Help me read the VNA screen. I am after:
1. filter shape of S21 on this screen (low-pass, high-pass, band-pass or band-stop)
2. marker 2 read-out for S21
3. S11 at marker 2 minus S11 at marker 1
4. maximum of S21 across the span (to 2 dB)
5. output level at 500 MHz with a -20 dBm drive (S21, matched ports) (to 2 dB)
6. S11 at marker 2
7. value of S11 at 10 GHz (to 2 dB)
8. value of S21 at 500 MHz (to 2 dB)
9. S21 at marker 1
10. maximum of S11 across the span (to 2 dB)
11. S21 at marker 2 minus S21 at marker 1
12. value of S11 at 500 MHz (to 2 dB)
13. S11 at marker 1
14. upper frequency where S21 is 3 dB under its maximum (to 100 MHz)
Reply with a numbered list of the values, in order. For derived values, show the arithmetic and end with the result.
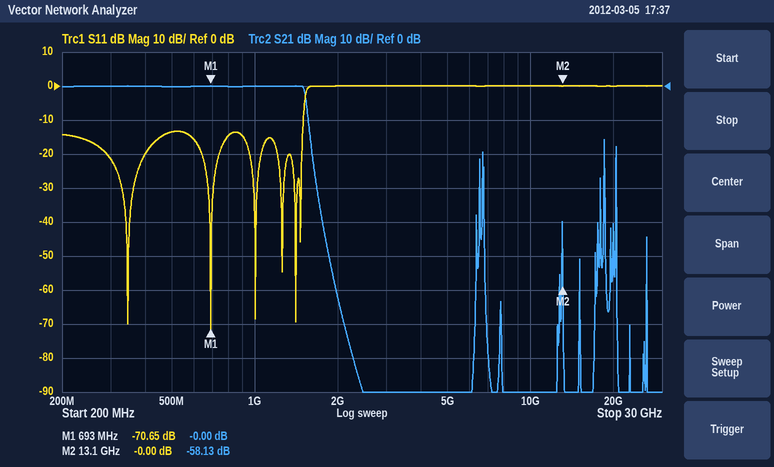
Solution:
1. low-pass
2. -58.13 dB
3. -0 − (-70.65) = 70.65 dB
4. 0 dB
5. -20 dBm + (0 dB) = -20 dBm
6. -0.00 dB
7. 0 dB
8. 0 dB
9. -0.00 dB
10. 0 dB
11. -58.13 − (-0) = -58.13 dB
12. -14 dB
13. -70.65 dB
14. 1.5 GHz
